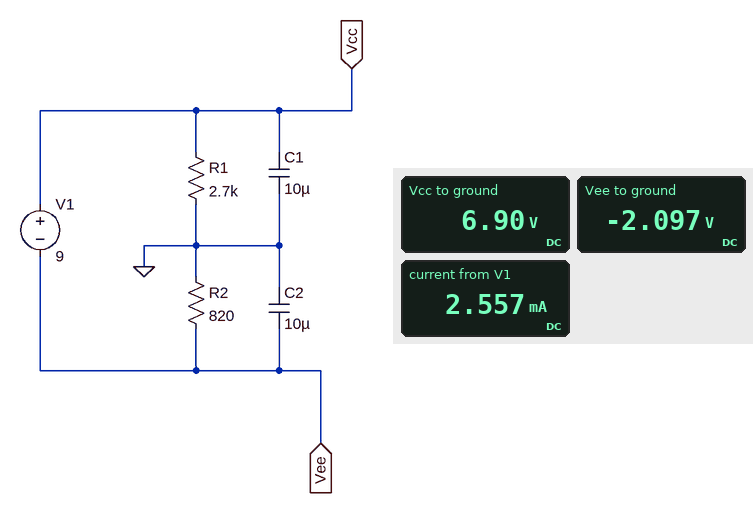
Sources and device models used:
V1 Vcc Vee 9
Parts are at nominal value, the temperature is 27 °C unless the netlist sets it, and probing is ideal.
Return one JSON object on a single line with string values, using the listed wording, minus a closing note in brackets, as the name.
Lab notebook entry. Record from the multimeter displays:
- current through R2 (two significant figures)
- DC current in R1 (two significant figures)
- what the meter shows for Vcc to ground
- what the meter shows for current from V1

{"current through R2": "2.6 mA", "DC current in R1": "2.6 mA", "what the meter shows for Vcc to ground": "6.90 V", "what the meter shows for current from V1": "2.557 mA"}
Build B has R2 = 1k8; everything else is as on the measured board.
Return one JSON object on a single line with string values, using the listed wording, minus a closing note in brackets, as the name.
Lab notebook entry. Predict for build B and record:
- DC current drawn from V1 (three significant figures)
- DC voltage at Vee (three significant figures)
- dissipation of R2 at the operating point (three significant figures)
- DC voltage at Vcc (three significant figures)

{"DC current drawn from V1": "2.00 mA", "DC voltage at Vee": "-3.60 V", "dissipation of R2 at the operating point": "7.20 mW", "DC voltage at Vcc": "5.40 V"}
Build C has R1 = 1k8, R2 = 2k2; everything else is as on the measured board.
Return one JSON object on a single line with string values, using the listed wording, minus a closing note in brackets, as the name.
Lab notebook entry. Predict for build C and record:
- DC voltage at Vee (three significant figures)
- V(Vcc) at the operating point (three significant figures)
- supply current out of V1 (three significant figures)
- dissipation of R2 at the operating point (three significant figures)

{"DC voltage at Vee": "-4.95 V", "V(Vcc) at the operating point": "4.05 V", "supply current out of V1": "2.25 mA", "dissipation of R2 at the operating point": "11.1 mW"}
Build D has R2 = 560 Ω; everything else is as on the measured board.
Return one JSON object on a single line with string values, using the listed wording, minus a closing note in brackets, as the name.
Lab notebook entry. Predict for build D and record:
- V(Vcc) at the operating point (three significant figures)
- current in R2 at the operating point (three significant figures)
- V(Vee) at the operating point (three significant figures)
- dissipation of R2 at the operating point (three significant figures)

{"V(Vcc) at the operating point": "7.45 V", "current in R2 at the operating point": "2.76 mA", "V(Vee) at the operating point": "-1.55 V", "dissipation of R2 at the operating point": "4.27 mW"}
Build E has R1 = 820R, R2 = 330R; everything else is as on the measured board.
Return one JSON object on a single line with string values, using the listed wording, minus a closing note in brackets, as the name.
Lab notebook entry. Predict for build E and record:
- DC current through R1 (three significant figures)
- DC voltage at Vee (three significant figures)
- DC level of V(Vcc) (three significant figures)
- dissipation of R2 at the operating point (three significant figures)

{"DC current through R1": "7.83 mA", "DC voltage at Vee": "-2.58 V", "DC level of V(Vcc)": "6.42 V", "dissipation of R2 at the operating point": "20.2 mW"}
